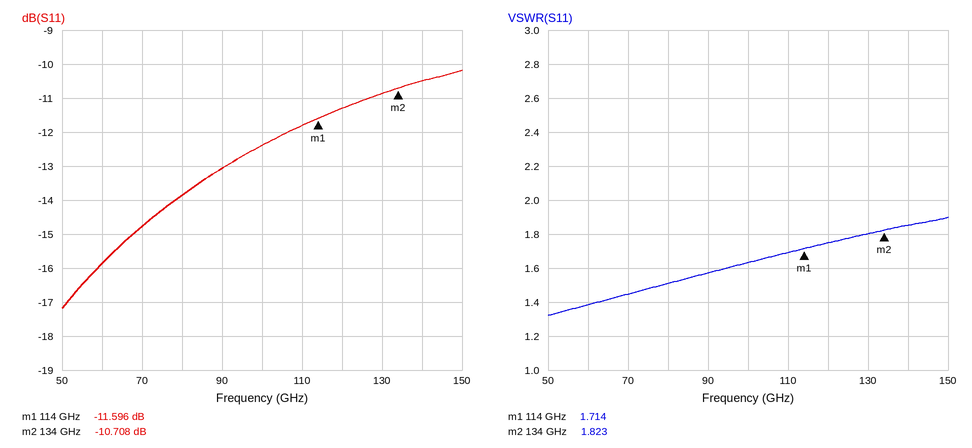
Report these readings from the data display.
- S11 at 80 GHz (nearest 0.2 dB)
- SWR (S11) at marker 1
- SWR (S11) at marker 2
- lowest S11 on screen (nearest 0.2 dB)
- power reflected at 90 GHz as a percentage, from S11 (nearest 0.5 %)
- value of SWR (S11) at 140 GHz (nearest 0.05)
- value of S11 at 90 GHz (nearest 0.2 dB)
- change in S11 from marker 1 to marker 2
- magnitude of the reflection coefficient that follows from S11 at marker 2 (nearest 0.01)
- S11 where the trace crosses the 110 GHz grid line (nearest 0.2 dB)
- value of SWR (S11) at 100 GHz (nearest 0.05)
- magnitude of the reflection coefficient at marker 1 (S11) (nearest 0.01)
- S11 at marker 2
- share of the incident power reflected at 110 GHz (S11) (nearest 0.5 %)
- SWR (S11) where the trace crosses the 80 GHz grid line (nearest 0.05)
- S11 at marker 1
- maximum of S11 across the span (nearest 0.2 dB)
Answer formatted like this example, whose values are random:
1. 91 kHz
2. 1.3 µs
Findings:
1. -13.8 dB
2. 1.714
3. 1.823
4. -17.2 dB
5. 5.0 %
6. 1.85
7. -13.0 dB
8. 0.888 dB
9. 0.29
10. -11.8 dB
11. 1.65
12. 0.26
13. -10.708 dB
14. 6.5 %
15. 1.50
16. -11.596 dB
17. -10.2 dB
